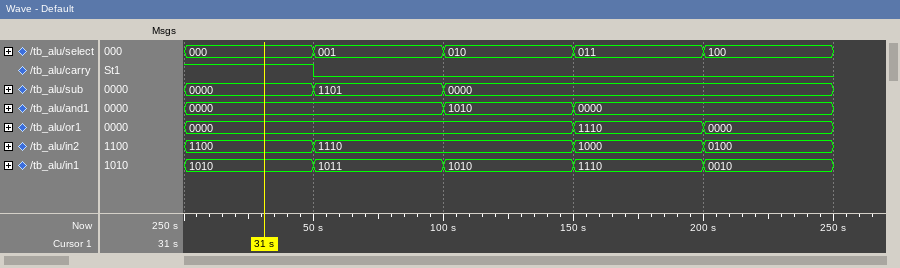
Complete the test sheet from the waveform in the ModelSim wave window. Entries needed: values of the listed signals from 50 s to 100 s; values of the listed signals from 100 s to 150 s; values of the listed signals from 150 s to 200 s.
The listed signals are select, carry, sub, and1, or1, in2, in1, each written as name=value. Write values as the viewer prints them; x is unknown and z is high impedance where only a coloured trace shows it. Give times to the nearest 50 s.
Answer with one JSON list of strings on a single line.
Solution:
["select=001, carry=0, sub=1101, and1=0000, or1=0000, in2=1110, in1=1011", "select=010, carry=0, sub=0000, and1=1010, or1=0000, in2=1110, in1=1010", "select=011, carry=0, sub=0000, and1=0000, or1=1110, in2=1000, in1=1110"]
